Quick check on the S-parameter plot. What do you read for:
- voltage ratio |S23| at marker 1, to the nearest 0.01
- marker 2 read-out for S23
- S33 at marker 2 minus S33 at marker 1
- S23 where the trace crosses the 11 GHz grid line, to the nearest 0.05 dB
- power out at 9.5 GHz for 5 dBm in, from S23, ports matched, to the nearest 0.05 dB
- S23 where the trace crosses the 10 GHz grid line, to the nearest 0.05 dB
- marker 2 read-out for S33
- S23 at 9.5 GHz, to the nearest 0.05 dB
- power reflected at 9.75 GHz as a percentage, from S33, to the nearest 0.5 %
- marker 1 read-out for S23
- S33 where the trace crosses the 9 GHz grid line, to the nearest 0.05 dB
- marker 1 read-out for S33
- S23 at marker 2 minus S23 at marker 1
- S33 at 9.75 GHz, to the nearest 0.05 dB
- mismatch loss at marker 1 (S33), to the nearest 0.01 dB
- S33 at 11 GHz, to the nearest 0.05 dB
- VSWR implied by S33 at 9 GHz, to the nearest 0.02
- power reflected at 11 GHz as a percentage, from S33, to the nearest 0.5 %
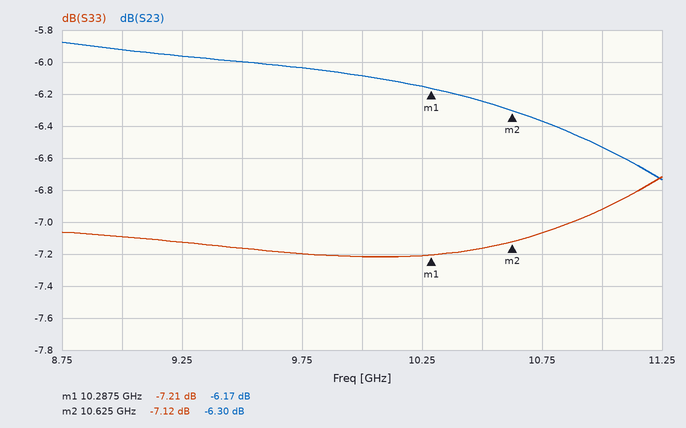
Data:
0.49
-6.30 dB
0.09 dB
-6.55 dB
-1.00 dBm
-6.10 dB
-7.12 dB
-6.00 dB
19.0 %
-6.17 dB
-7.10 dB
-7.21 dB
-0.13 dB
-7.20 dB
0.92 dB
-6.90 dB
2.58
20.5 %
